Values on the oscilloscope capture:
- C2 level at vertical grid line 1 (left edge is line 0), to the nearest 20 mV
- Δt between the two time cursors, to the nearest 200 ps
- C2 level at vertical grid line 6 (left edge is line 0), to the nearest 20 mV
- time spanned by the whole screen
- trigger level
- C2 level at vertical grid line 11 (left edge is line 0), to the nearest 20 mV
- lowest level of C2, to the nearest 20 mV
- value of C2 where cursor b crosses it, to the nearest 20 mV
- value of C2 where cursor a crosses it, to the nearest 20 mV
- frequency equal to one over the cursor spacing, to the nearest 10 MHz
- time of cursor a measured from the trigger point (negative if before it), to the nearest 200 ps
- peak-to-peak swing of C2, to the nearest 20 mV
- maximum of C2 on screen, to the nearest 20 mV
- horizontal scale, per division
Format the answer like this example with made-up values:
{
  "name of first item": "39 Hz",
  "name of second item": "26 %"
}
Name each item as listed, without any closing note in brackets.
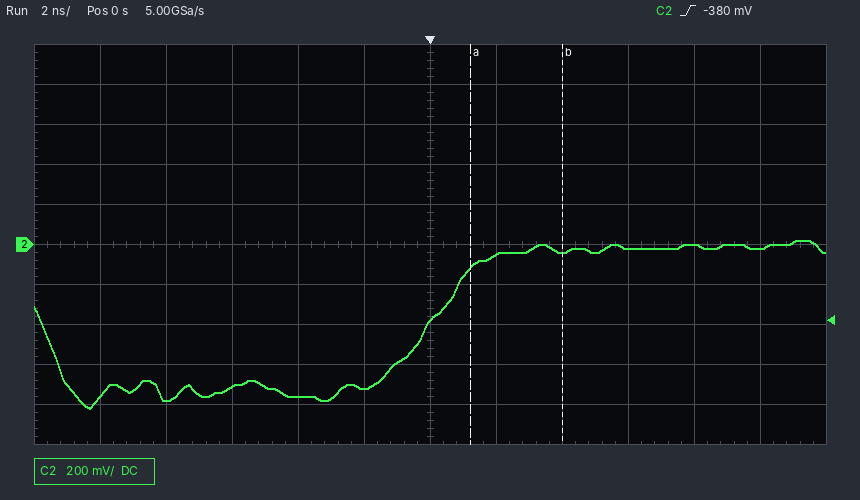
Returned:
{
  "C2 level at vertical grid line 1 (left edge is line 0), to the nearest 20 mV": "-760 mV",
  "Δt between the two time cursors, to the nearest 200 ps": "2.8 ns",
  "C2 level at vertical grid line 6 (left edge is line 0), to the nearest 20 mV": "-380 mV",
  "time spanned by the whole screen": "24 ns",
  "trigger level": "-380 mV",
  "C2 level at vertical grid line 11 (left edge is line 0), to the nearest 20 mV": "-20 mV",
  "lowest level of C2, to the nearest 20 mV": "-820 mV",
  "value of C2 where cursor b crosses it, to the nearest 20 mV": "-40 mV",
  "value of C2 where cursor a crosses it, to the nearest 20 mV": "-120 mV",
  "frequency equal to one over the cursor spacing, to the nearest 10 MHz": "360 MHz",
  "time of cursor a measured from the trigger point (negative if before it), to the nearest 200 ps": "+1.2 ns",
  "peak-to-peak swing of C2, to the nearest 20 mV": "840 mV",
  "maximum of C2 on screen, to the nearest 20 mV": "20 mV",
  "horizontal scale, per division": "2 ns"
}
